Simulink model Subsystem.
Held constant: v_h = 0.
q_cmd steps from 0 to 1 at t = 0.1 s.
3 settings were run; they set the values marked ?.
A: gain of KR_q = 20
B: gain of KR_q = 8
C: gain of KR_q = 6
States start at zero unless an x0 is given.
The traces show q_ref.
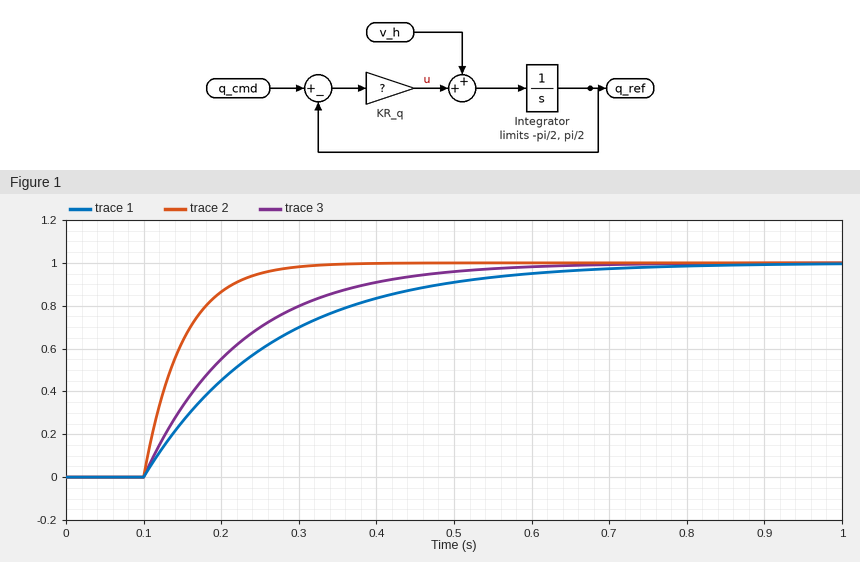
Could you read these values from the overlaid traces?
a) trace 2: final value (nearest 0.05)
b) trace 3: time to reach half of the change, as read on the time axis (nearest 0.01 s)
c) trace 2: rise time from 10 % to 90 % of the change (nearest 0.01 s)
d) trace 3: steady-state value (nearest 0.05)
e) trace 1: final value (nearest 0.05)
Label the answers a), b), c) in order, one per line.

a) 1.00
b) 0.19 s
c) 0.11 s
d) 1.00
e) 1.00
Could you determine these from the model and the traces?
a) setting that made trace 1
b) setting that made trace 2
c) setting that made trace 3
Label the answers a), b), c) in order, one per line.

a) C
b) A
c) B
